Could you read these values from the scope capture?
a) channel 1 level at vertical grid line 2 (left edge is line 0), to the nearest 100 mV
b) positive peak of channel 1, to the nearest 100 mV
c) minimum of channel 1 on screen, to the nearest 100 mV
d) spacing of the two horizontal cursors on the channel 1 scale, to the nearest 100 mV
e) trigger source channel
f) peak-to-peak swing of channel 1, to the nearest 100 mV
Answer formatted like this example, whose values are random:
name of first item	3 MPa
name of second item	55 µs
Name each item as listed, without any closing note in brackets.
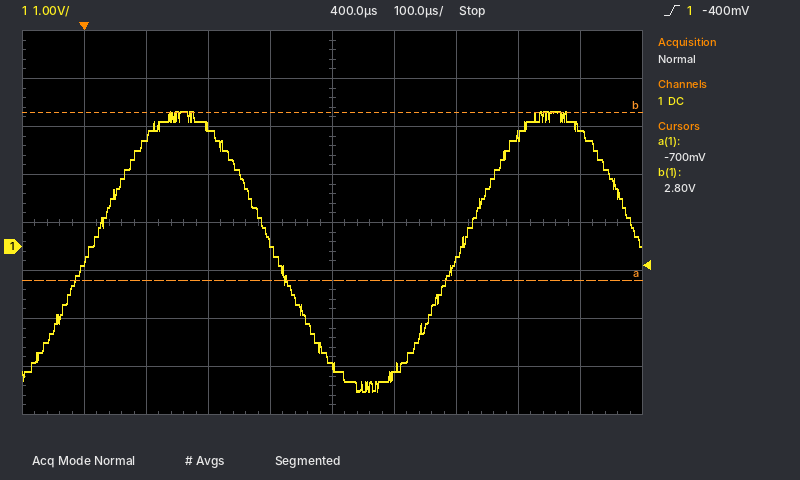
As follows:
channel 1 level at vertical grid line 2 (left edge is line 0), to the nearest 100 mV	2.3 V
positive peak of channel 1, to the nearest 100 mV	2.8 V
minimum of channel 1 on screen, to the nearest 100 mV	-3.0 V
spacing of the two horizontal cursors on the channel 1 scale, to the nearest 100 mV	3.5 V
trigger source channel	channel 1
peak-to-peak swing of channel 1, to the nearest 100 mV	5.8 V
